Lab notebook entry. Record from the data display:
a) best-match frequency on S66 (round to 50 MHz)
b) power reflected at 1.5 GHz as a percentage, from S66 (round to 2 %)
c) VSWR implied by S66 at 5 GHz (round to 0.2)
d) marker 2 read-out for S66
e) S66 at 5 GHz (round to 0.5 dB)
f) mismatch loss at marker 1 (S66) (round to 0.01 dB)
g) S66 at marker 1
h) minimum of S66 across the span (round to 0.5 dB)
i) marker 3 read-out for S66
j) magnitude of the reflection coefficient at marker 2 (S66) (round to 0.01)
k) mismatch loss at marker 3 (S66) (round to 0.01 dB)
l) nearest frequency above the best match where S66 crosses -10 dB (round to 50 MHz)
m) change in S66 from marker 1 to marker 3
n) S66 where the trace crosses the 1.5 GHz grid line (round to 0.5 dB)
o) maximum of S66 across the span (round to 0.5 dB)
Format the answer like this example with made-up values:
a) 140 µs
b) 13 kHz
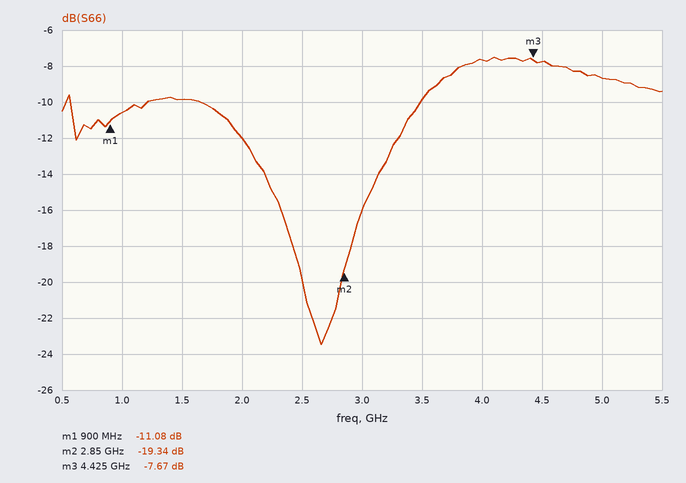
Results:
a) 2.65 GHz
b) 10 %
c) 2.2
d) -19.34 dB
e) -8.5 dB
f) 0.35 dB
g) -11.08 dB
h) -23.5 dB
i) -7.67 dB
j) 0.11
k) 0.81 dB
l) 3.50 GHz
m) 3.41 dB
n) -10.0 dB
o) -7.5 dB
